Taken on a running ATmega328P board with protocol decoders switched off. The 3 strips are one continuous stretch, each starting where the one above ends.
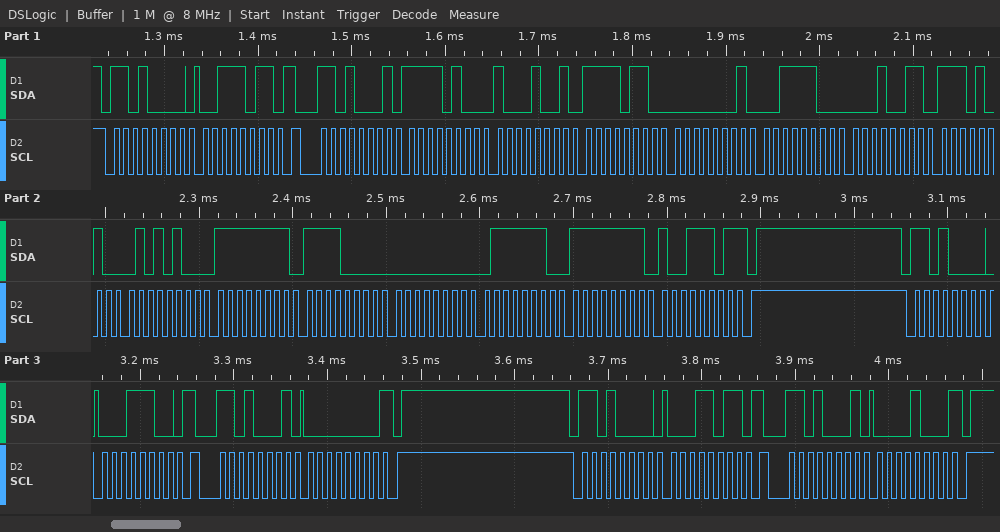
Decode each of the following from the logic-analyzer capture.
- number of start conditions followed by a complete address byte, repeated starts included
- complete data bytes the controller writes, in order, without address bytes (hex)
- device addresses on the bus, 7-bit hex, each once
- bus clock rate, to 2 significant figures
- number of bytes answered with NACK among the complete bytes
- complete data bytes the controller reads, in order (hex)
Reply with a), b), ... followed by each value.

a) 6
b) 3B 1C 1B
c) 0x68
d) 100 kHz
e) 3
f) F4 89 F6 01 3C 13 EA 54 FF F0 00 7E FF 9D 00 08
